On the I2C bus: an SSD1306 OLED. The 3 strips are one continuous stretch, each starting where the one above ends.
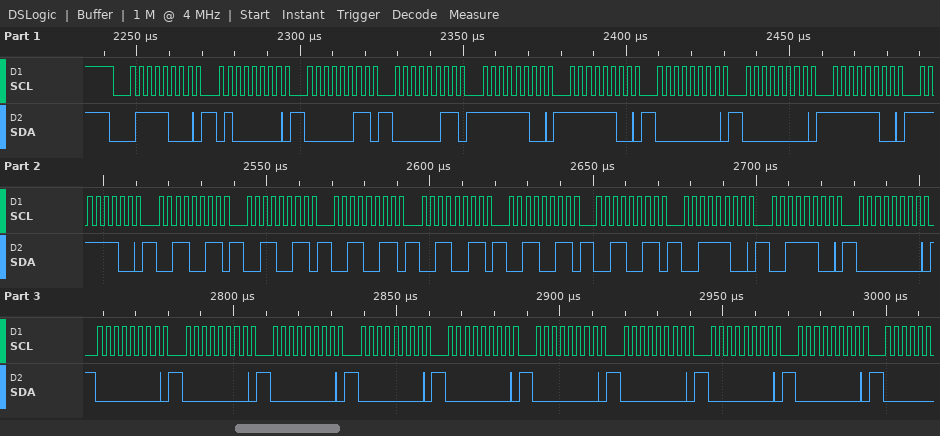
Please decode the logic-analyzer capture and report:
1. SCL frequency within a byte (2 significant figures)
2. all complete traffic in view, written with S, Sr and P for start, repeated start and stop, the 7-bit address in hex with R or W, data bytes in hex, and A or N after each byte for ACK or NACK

400 kHz
S 3CW A 40 A 03 A 03 A FC A FC A 00 A 00 A FC A FC A 33 A 33 A 33 A 33 A 33 A 33 A 3C A 3C A 00 A 00 A 00 A 00 A 00 A 00 A 00 A 00 A 00 A 00 A
